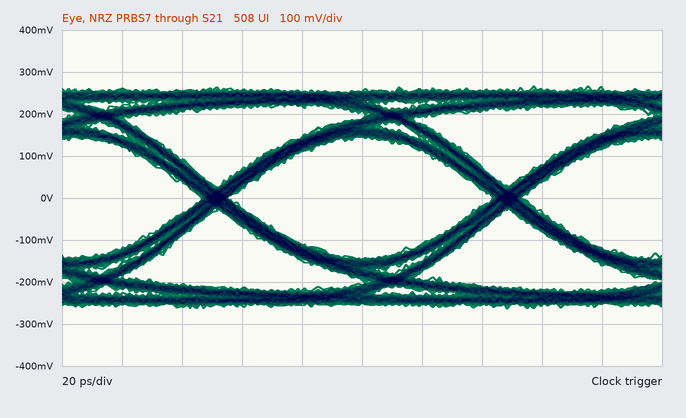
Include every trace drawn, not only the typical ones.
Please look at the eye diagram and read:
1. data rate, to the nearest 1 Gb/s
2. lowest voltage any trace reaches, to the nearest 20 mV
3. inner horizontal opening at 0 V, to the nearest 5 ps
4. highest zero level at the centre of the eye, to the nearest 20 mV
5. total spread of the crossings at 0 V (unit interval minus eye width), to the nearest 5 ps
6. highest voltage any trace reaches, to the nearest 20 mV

10 Gb/s
-260 mV
90 ps
-140 mV
10 ps
260 mV
